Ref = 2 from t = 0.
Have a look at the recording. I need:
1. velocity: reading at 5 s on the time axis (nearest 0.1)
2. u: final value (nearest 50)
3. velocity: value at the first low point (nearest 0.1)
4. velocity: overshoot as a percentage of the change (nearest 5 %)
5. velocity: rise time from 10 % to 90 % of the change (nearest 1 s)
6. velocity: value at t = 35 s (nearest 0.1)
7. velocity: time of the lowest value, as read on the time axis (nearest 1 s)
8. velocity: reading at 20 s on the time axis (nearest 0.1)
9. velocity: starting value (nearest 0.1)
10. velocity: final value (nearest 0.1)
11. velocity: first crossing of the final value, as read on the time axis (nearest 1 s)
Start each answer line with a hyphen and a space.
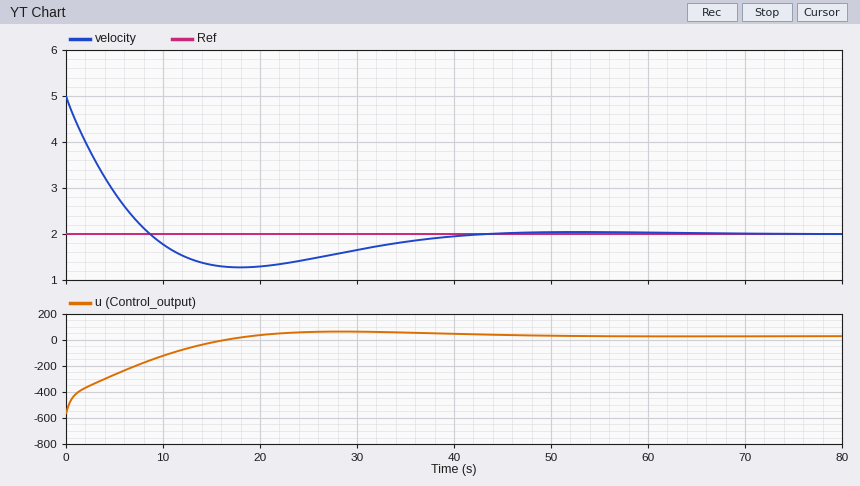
- 2.9
- 50
- 1.3
- 25 %
- 7 s
- 1.8
- 18 s
- 1.3
- 5.0
- 2.0
- 9 s
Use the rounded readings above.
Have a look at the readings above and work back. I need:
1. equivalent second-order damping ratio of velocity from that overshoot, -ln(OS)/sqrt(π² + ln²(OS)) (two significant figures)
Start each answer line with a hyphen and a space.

- 0.40
